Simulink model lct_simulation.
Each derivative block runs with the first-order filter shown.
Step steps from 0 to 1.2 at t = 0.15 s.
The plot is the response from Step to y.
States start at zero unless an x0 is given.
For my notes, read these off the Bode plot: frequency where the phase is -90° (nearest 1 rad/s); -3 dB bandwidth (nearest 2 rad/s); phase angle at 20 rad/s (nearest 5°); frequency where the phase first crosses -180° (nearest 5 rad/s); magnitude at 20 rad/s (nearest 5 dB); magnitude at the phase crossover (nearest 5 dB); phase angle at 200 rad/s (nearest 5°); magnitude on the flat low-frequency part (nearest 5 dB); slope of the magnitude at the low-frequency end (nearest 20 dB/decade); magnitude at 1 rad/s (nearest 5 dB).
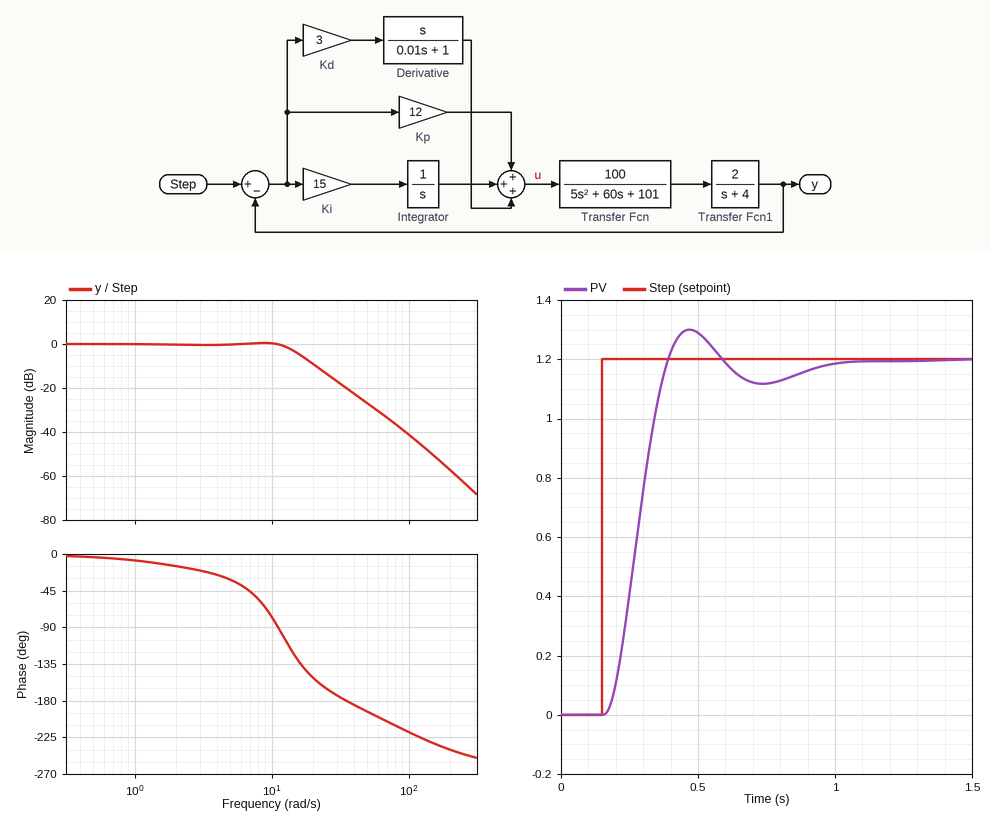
11 rad/s
14 rad/s
-150°
35 rad/s
-10 dB
-20 dB
-240°
0 dB
0 dB/decade
0 dB
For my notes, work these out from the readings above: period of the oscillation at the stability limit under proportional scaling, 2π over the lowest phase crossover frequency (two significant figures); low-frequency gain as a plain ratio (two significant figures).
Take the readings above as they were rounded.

0.18 s
1.0
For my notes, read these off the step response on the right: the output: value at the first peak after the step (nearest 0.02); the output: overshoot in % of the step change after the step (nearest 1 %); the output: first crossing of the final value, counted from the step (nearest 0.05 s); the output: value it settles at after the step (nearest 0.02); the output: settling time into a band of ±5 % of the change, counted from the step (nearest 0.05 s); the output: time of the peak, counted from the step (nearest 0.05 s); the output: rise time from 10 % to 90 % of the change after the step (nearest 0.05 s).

1.30
8 %
0.25 s
1.20
0.70 s
0.30 s
0.15 s
